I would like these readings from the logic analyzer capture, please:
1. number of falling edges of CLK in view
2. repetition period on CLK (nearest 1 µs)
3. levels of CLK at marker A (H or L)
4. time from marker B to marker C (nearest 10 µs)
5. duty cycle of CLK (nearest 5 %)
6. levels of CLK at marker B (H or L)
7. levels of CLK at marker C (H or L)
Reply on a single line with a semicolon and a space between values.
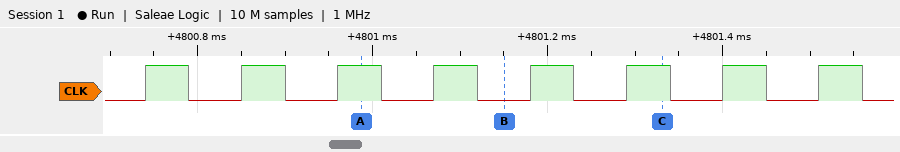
8; 110 µs; CLK=H; 180 µs; 45 %; CLK=L; CLK=H
